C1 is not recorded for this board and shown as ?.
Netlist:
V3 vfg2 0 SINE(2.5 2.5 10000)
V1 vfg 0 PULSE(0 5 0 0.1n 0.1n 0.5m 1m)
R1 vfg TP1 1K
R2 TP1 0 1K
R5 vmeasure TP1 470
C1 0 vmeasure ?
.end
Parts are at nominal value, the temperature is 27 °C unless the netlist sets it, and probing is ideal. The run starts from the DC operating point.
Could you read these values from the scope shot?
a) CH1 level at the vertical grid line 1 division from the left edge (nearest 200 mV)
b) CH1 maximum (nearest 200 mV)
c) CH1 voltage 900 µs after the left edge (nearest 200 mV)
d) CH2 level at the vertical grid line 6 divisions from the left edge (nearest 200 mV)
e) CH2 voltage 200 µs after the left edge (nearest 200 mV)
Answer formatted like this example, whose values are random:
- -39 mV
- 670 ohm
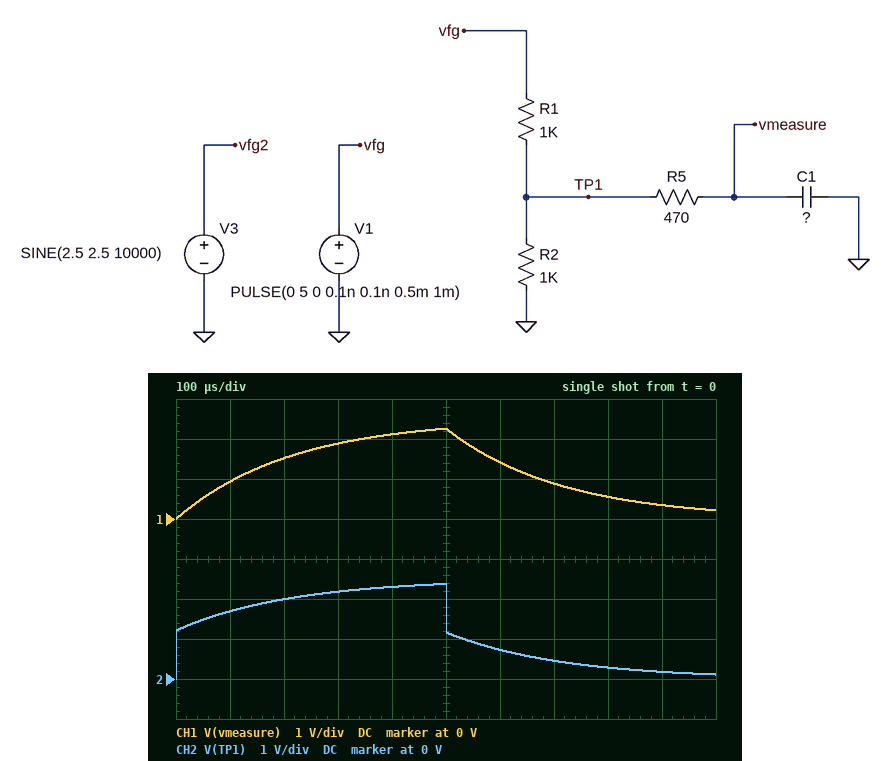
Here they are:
- 1.0 V
- 2.2 V
- 400 mV
- 800 mV
- 2.0 V
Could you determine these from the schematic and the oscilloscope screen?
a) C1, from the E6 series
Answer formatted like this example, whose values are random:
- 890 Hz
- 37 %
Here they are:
- 220 nF
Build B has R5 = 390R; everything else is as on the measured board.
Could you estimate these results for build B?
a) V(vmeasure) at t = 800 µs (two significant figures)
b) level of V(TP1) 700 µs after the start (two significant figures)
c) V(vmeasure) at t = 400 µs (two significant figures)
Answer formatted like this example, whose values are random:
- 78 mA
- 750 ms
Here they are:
- 500 mV
- 470 mV
- 2.2 V
